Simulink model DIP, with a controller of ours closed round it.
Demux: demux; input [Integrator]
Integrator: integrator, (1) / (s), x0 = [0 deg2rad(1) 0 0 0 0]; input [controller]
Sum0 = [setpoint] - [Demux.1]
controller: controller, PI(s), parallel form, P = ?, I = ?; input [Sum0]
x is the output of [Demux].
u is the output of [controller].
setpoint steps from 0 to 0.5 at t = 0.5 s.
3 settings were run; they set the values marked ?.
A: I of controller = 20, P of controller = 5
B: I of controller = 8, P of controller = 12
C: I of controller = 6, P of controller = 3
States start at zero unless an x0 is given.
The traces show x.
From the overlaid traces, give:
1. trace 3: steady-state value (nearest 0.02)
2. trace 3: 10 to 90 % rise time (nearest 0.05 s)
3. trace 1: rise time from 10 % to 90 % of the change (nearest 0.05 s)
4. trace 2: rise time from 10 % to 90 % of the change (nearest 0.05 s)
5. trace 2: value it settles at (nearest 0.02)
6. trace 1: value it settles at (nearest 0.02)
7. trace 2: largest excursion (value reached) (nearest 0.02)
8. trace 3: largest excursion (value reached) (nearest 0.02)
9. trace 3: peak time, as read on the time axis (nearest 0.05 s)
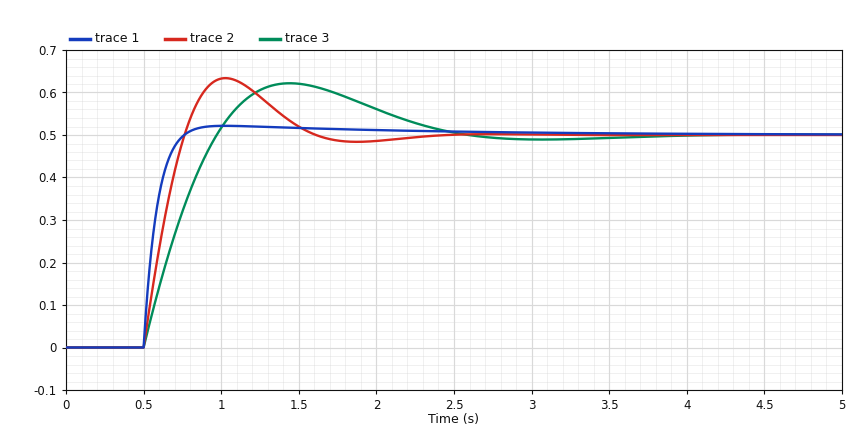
0.50
0.35 s
0.15 s
0.20 s
0.50
0.50
0.64
0.62
1.45 s
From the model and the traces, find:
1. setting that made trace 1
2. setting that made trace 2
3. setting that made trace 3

B
A
C
